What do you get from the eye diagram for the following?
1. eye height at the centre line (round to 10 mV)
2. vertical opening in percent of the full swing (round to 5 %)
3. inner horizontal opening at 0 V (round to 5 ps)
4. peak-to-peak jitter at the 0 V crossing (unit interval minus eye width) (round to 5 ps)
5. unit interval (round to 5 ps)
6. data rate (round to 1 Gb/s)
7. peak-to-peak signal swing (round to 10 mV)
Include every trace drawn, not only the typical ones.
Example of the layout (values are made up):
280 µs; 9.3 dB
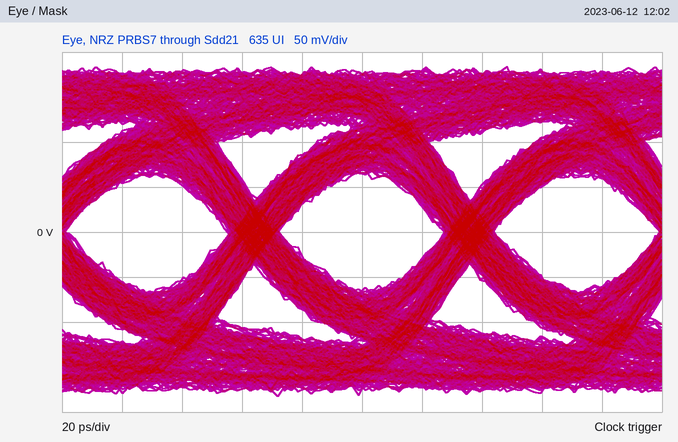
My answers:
130 mV; 35 %; 55 ps; 15 ps; 70 ps; 14 Gb/s; 370 mV
